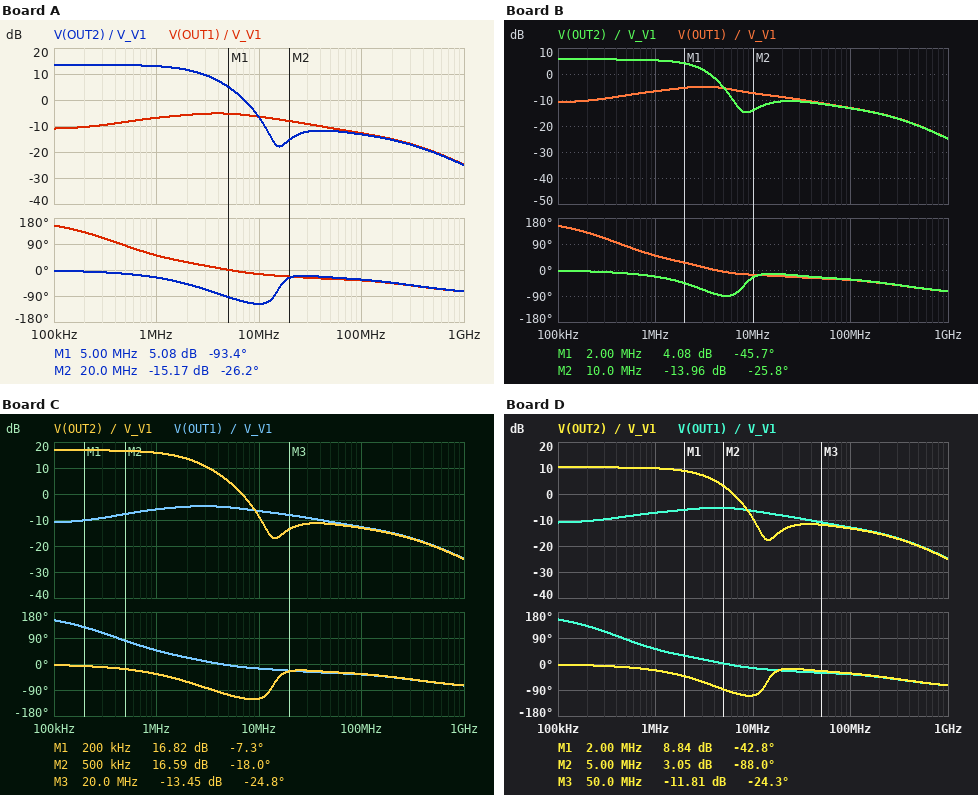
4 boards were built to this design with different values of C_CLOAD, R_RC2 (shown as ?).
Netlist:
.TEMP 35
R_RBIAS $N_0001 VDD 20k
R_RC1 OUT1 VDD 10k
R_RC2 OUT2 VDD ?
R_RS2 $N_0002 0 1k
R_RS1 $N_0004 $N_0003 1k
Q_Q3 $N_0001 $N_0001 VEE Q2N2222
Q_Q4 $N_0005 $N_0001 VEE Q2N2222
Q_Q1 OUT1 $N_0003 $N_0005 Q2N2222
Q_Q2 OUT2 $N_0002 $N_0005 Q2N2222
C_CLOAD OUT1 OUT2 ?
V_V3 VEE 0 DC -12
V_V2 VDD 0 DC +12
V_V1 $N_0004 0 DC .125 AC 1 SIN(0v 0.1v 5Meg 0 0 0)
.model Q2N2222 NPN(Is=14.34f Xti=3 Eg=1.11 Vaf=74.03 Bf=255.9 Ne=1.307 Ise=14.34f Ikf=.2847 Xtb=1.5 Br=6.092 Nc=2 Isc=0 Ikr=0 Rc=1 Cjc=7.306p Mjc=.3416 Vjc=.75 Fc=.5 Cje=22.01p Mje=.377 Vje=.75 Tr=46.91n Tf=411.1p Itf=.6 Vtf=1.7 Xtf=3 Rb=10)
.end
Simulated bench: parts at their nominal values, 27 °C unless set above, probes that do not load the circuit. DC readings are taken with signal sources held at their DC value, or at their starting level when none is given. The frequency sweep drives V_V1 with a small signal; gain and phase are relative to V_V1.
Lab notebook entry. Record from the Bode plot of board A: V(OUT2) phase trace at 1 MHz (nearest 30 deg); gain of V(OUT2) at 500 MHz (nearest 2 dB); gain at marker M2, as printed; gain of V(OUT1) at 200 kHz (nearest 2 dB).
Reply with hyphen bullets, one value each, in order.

- -30 deg
- -20 dB
- -15.17 dB
- -10 dB
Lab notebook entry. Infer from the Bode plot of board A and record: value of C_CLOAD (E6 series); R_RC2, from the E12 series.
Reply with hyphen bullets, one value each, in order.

- 2.2 pF
- 8.2 kΩ
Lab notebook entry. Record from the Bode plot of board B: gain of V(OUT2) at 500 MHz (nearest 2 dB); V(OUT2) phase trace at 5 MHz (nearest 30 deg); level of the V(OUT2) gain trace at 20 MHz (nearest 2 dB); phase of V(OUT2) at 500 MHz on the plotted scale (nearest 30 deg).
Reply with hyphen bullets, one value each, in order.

- -20 dB
- -90 deg
- -10 dB
- -60 deg
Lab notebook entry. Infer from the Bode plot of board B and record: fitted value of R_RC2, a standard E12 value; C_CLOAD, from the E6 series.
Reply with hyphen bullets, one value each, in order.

- 3.3 kΩ
- 15 pF
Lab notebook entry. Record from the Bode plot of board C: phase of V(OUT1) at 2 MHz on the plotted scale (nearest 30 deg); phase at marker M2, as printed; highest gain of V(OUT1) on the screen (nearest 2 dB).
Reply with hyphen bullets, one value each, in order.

- 30 deg
- -18.0 deg
- -4 dB
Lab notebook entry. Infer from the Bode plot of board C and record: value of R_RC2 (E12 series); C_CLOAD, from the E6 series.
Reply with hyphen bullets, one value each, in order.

- 12 kΩ
- 3.3 pF
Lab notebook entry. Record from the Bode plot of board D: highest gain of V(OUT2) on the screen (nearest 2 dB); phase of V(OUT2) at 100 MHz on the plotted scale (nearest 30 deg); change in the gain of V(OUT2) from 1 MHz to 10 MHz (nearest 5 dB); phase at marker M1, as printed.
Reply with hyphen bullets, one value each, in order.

- 10 dB
- -30 deg
- -20 dB
- -42.8 deg
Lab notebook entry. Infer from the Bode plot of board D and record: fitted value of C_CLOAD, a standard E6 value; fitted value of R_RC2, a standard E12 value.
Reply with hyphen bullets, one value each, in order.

- 3.3 pF
- 5.6 kΩ
